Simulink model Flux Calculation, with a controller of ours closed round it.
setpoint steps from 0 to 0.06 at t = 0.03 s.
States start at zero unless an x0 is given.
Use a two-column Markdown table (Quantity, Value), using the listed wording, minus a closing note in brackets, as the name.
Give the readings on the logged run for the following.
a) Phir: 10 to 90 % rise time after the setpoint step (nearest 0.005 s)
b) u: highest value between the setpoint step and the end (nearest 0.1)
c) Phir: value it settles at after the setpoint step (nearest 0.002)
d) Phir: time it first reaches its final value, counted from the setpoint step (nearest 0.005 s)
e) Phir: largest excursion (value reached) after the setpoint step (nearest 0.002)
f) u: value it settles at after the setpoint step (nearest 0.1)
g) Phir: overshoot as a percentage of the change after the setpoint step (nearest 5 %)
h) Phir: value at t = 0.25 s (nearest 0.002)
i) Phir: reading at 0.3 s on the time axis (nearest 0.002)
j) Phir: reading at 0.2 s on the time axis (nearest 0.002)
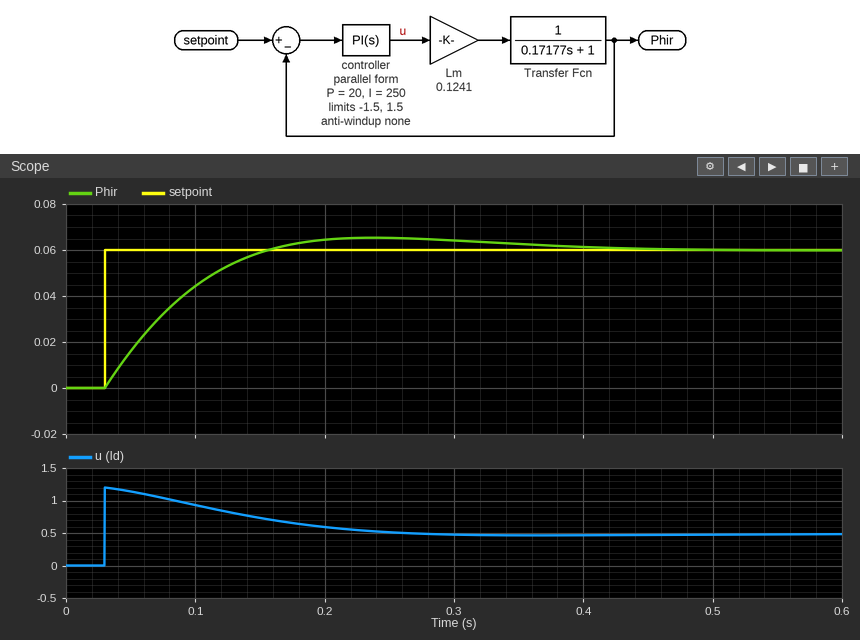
| Quantity | Value |
|---|---|
| Phir: 10 to 90 % rise time after the setpoint step | 0.090 s |
| u: highest value between the setpoint step and the end | 1.2 |
| Phir: value it settles at after the setpoint step | 0.060 |
| Phir: time it first reaches its final value, counted from the setpoint step | 0.125 s |
| Phir: largest excursion (value reached) after the setpoint step | 0.066 |
| u: value it settles at after the setpoint step | 0.5 |
| Phir: overshoot as a percentage of the change after the setpoint step | 10 % |
| Phir: value at t = 0.25 s | 0.066 |
| Phir: reading at 0.3 s on the time axis | 0.064 |
| Phir: reading at 0.2 s on the time axis | 0.064 |
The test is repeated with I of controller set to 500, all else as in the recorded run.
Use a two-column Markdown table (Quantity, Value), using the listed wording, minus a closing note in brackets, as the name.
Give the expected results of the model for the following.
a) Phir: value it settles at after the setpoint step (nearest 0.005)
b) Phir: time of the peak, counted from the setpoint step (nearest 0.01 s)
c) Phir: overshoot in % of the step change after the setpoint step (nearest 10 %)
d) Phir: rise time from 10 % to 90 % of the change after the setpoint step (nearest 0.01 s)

| Quantity | Value |
|---|---|
| Phir: value it settles at after the setpoint step | 0.060 |
| Phir: time of the peak, counted from the setpoint step | 0.14 s |
| Phir: overshoot in % of the step change after the setpoint step | 20 % |
| Phir: rise time from 10 % to 90 % of the change after the setpoint step | 0.06 s |
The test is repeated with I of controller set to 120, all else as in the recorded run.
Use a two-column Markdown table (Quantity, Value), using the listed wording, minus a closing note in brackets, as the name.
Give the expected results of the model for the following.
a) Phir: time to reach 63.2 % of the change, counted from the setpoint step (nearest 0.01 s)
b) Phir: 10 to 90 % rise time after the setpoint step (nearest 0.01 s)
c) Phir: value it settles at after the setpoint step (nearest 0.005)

| Quantity | Value |
|---|---|
| Phir: time to reach 63.2 % of the change, counted from the setpoint step | 0.07 s |
| Phir: 10 to 90 % rise time after the setpoint step | 0.15 s |
| Phir: value it settles at after the setpoint step | 0.060 |
